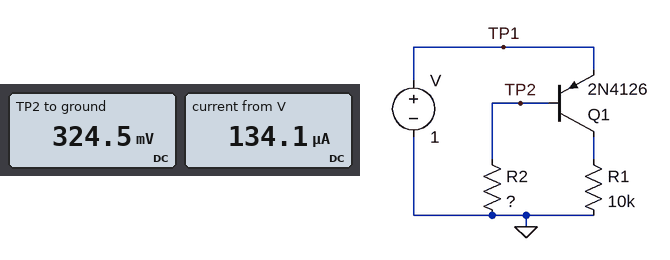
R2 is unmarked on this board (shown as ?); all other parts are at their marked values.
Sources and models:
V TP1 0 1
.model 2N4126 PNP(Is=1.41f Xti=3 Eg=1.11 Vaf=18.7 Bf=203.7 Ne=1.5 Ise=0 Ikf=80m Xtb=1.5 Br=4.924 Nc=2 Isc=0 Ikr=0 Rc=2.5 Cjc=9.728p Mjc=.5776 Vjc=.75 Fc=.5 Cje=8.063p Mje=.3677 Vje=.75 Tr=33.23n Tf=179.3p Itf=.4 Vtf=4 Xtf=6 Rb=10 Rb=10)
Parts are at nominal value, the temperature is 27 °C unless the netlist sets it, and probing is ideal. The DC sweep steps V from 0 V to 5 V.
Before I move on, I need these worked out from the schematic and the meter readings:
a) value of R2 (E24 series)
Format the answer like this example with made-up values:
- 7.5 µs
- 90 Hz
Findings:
- 9.1 kΩ
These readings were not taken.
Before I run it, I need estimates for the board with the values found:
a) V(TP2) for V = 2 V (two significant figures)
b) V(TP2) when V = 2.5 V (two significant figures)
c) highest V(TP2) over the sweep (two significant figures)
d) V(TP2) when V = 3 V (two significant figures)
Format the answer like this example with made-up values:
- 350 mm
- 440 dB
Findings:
- 1.3 V
- 1.8 V
- 4.3 V
- 2.3 V
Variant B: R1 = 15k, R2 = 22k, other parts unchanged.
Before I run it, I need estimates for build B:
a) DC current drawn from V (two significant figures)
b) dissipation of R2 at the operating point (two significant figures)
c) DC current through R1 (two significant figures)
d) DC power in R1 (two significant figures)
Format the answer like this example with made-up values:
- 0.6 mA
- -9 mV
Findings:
- 81 µA
- 5.3 µW
- 65 µA
- 64 µW
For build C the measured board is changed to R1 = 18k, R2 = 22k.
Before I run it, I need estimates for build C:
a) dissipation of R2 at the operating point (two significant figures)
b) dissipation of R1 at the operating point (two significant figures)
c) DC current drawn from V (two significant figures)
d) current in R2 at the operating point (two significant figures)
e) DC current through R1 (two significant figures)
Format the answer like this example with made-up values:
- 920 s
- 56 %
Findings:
- 5.4 µW
- 54 µW
- 70 µA
- 16 µA
- 55 µA
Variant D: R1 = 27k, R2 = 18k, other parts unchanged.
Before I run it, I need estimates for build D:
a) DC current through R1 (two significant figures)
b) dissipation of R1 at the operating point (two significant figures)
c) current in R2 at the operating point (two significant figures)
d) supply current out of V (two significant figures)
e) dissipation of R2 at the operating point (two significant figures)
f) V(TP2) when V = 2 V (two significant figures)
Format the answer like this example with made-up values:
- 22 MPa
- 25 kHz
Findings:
- 37 µA
- 36 µW
- 19 µA
- 56 µA
- 6.6 µW
- 1.3 V
